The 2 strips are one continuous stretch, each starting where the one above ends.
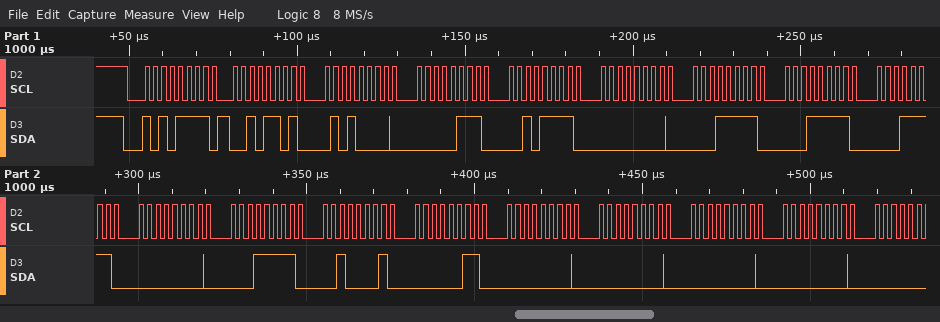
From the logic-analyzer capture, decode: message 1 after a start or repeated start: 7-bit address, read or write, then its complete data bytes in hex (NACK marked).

0x57 read: 2D 50 07 2F 00 1F 1F 1F 00 1F 21 03 00 00 00 00
